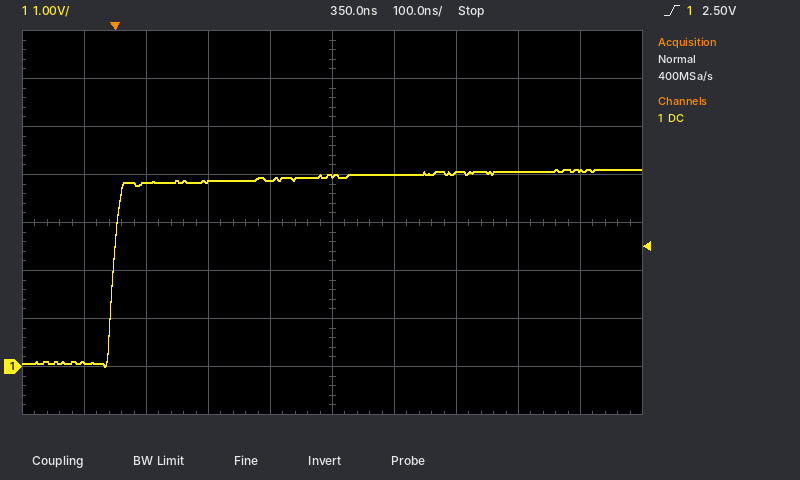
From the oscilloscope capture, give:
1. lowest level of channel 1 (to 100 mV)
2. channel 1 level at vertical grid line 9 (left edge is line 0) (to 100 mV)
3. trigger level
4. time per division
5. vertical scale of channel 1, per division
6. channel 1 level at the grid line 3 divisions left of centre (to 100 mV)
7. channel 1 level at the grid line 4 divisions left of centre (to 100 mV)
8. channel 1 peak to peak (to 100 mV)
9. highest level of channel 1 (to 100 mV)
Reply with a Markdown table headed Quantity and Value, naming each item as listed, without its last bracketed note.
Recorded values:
| Quantity | Value |
|---|---|
| lowest level of channel 1 | 0.0 V |
| channel 1 level at vertical grid line 9 (left edge is line 0) | 4.1 V |
| trigger level | 2.50 V |
| time per division | 100 ns |
| vertical scale of channel 1, per division | 1 V |
| channel 1 level at the grid line 3 divisions left of centre | 3.8 V |
| channel 1 level at the grid line 4 divisions left of centre | 100 mV |
| channel 1 peak to peak | 4.1 V |
| highest level of channel 1 | 4.1 V |
